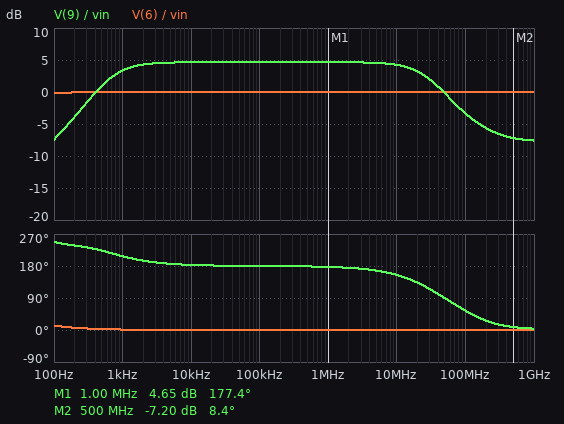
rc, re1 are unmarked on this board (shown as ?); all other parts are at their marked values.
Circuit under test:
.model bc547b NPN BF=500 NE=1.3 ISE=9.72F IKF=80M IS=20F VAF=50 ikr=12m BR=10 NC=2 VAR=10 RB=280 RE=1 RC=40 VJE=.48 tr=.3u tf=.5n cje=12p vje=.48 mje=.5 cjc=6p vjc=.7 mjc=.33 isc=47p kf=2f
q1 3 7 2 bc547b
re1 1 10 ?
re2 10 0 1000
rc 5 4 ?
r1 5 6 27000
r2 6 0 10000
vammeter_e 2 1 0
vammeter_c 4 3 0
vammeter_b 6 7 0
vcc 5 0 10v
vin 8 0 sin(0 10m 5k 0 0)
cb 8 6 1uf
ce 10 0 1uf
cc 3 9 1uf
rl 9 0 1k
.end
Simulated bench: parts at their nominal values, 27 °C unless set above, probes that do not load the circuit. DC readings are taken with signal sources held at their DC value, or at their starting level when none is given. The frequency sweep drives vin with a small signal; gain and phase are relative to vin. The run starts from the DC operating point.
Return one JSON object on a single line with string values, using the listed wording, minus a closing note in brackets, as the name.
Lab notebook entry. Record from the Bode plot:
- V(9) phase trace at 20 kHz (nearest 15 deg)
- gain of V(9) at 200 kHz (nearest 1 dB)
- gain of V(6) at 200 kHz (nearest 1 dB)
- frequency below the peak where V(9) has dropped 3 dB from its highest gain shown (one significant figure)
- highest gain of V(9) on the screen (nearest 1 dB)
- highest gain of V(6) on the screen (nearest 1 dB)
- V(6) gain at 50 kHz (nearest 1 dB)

{"V(9) phase trace at 20 kHz": "180 deg", "gain of V(9) at 200 kHz": "5 dB", "gain of V(6) at 200 kHz": "0 dB", "frequency below the peak where V(9) has dropped 3 dB from its highest gain shown": "600 Hz", "highest gain of V(9) on the screen": "5 dB", "highest gain of V(6) on the screen": "0 dB", "V(6) gain at 50 kHz": "0 dB"}
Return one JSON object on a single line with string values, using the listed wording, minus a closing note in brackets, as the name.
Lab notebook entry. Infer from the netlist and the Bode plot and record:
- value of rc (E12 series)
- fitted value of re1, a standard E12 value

{"value of rc": "1.5 kΩ", "fitted value of re1, a standard E12 value": "330 Ω"}
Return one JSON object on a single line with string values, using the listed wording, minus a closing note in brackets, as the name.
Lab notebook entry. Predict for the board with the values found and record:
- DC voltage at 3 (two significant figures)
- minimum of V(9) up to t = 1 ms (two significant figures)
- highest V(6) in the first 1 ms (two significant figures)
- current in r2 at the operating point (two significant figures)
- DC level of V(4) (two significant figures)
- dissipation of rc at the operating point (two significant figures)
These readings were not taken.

{"DC voltage at 3": "7.7 V", "minimum of V(9) up to t = 1 ms": "-17 mV", "highest V(6) in the first 1 ms": "2.7 V", "current in r2 at the operating point": "270 µA", "DC level of V(4)": "7.7 V", "dissipation of rc at the operating point": "3.4 mW"}
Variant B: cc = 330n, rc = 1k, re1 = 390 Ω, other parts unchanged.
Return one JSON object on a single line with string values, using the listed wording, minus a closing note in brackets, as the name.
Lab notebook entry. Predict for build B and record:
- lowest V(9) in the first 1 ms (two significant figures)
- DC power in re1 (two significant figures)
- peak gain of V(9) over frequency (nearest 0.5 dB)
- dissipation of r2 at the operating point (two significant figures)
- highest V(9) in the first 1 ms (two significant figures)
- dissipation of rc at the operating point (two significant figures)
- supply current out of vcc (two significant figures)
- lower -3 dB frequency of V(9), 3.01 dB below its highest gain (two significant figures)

{"lowest V(9) in the first 1 ms": "-12 mV", "DC power in re1": "820 µW", "peak gain of V(9) over frequency": "1.5 dB", "dissipation of r2 at the operating point": "710 µW", "highest V(9) in the first 1 ms": "13 mV", "dissipation of rc at the operating point": "2.1 mW", "supply current out of vcc": "1.7 mA", "lower -3 dB frequency of V(9), 3.01 dB below its highest gain": "600 Hz"}
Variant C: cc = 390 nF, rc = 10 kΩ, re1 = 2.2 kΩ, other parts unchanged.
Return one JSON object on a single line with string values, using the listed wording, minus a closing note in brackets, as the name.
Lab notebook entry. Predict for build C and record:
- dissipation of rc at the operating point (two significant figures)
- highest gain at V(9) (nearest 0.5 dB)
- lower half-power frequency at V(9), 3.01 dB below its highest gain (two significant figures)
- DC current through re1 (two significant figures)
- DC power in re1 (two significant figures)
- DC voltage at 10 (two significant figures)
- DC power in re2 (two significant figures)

{"dissipation of rc at the operating point": "4.1 mW", "highest gain at V(9)": "-3.0 dB", "lower half-power frequency at V(9), 3.01 dB below its highest gain": "12 MHz", "DC current through re1": "640 µA", "DC power in re1": "910 µW", "DC voltage at 10": "640 mV", "DC power in re2": "410 µW"}
